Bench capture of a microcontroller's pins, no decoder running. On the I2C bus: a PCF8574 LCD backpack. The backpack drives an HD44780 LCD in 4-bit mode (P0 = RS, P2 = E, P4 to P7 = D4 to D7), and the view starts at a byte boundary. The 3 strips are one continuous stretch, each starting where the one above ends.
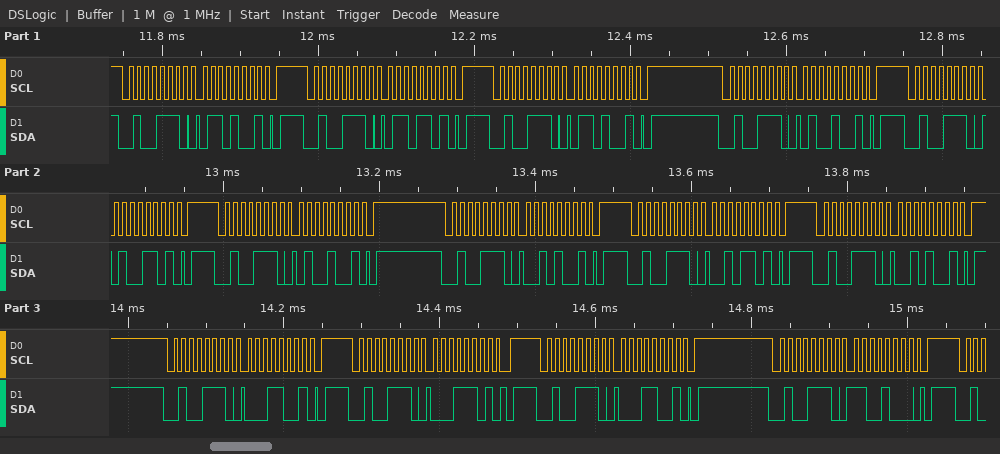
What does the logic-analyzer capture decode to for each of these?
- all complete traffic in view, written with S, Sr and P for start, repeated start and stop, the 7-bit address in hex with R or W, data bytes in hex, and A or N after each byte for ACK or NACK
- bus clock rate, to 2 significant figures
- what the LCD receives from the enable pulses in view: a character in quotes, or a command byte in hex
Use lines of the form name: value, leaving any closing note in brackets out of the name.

all complete traffic in view, written with S, Sr and P for start, repeated start and stop, the 7-bit address in hex with R or W, data bytes in hex, and A or N after each byte for ACK or NACK: S 27W A 69 A P S 27W A 6D A P S 27W A 69 A P S 27W A 49 A P S 27W A 4D A P S 27W A 49 A P S 27W A 29 A P S 27W A 2D A P S 27W A 29 A P S 27W A 19 A P S 27W A 1D A P S 27W A 19 A P S 27W A C8 A P
bus clock rate, to 2 significant figures: 100 kHz
what the LCD receives from the enable pulses in view: a character in quotes, or a command byte in hex: 'd' '!'
